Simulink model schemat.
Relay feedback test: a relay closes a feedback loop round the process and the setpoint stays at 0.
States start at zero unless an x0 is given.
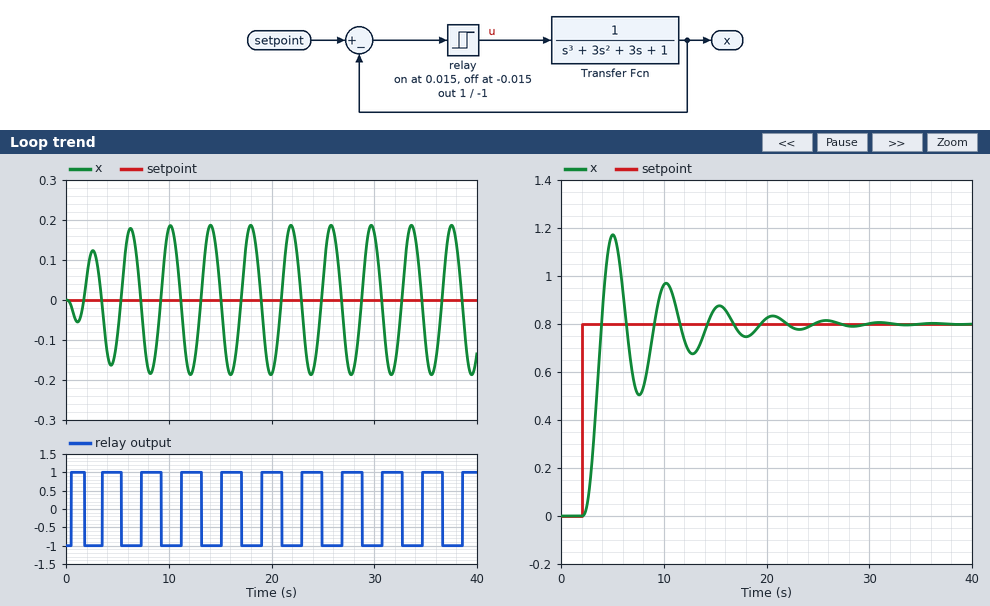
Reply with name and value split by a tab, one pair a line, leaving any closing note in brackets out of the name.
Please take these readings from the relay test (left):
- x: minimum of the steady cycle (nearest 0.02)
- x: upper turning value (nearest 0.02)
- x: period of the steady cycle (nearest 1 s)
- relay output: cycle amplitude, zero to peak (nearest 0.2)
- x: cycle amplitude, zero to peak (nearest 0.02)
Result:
x: minimum of the steady cycle	-0.18
x: upper turning value	0.18
x: period of the steady cycle	4 s
relay output: cycle amplitude, zero to peak	1.0
x: cycle amplitude, zero to peak	0.18
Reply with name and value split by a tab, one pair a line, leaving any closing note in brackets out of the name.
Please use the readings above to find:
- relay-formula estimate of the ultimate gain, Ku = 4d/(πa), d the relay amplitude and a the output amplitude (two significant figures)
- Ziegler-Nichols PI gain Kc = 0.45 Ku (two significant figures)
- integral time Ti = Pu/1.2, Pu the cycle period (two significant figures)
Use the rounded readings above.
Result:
relay-formula estimate of the ultimate gain, Ku = 4d/(πa), d the relay amplitude and a the output amplitude	7.1
Ziegler-Nichols PI gain Kc = 0.45 Ku	3.2
integral time Ti = Pu/1.2, Pu the cycle period	3.3 s
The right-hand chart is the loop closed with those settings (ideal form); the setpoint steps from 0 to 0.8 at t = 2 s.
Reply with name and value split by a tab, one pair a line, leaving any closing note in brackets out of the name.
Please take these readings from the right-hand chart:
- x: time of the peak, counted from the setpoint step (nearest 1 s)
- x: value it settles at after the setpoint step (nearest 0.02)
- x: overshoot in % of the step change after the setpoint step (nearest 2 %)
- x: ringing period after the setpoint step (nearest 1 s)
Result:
x: time of the peak, counted from the setpoint step	3 s
x: value it settles at after the setpoint step	0.80
x: overshoot in % of the step change after the setpoint step	46 %
x: ringing period after the setpoint step	5 s
